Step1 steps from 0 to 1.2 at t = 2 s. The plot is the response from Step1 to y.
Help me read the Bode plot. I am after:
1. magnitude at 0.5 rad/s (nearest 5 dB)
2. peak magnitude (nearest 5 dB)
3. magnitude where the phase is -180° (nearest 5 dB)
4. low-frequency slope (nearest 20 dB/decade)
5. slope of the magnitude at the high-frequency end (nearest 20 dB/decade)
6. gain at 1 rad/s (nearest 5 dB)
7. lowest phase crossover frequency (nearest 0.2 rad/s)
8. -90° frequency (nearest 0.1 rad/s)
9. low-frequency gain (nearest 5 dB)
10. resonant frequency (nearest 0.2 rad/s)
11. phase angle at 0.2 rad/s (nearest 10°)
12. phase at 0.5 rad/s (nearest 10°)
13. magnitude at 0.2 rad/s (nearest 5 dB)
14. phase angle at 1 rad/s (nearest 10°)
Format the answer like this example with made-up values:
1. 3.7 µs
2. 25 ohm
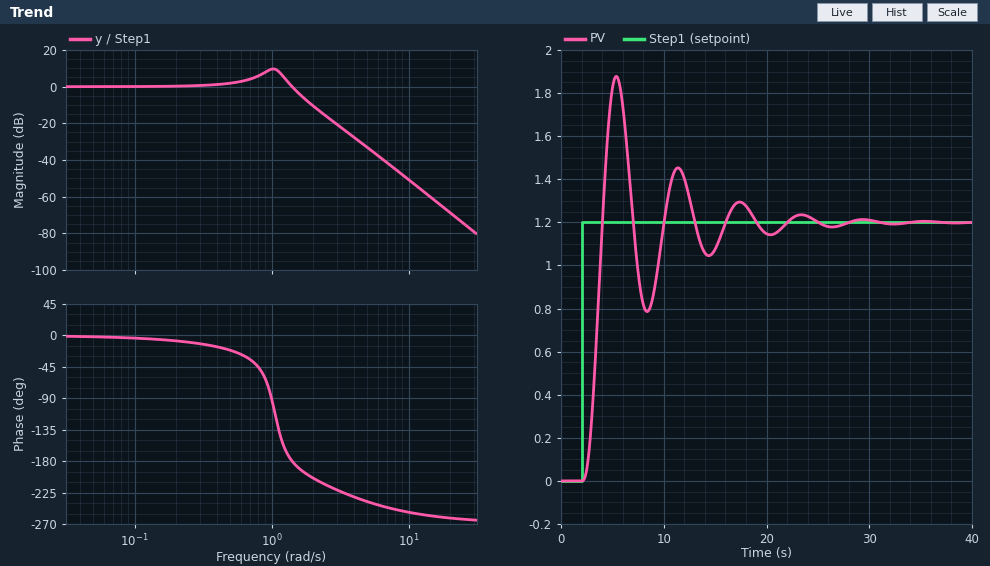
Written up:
1. 0 dB
2. 10 dB
3. 0 dB
4. 0 dB/decade
5. -60 dB/decade
6. 10 dB
7. 1.4 rad/s
8. 1.0 rad/s
9. 0 dB
10. 1.0 rad/s
11. -10°
12. -20°
13. 0 dB
14. -90°
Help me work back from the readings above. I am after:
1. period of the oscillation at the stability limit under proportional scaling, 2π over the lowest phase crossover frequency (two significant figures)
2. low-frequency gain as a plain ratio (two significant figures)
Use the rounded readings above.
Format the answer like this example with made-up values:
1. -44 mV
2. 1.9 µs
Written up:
1. 4.5 s
2. 1.0
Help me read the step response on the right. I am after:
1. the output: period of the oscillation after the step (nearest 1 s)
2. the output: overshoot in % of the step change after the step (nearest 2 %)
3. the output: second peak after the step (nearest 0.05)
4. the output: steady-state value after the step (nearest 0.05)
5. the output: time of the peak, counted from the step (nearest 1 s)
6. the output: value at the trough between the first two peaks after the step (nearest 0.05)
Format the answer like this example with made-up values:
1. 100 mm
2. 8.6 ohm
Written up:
1. 6 s
2. 56 %
3. 1.45
4. 1.20
5. 3 s
6. 0.80
